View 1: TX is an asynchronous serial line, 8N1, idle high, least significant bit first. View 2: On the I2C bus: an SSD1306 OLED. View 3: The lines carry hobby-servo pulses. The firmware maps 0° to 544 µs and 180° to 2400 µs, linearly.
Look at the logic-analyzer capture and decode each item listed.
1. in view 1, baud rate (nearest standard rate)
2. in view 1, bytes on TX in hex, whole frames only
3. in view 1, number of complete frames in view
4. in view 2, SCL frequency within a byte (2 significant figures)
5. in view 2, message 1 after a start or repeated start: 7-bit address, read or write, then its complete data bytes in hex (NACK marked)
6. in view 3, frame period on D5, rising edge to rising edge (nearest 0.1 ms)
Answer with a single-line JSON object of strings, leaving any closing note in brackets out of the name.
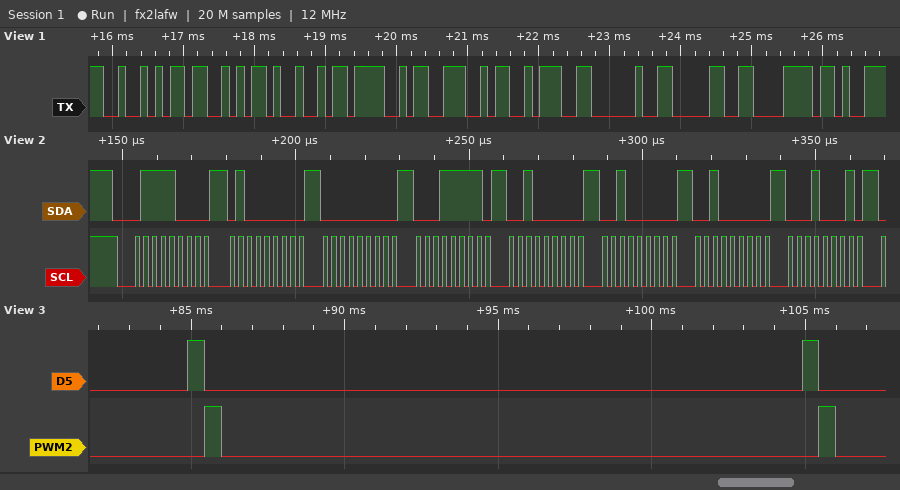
{"in view 1, baud rate": "9600 baud", "in view 1, bytes on TX in hex, whole frames only": "0x52 0x53 0x49 0x4F 0x4E 0x3A 0x20 0x30 0x78", "in view 1, number of complete frames in view": "9", "in view 2, SCL frequency within a byte": "400 kHz", "in view 2, message 1 after a start or repeated start: 7-bit address, read or write, then its complete data bytes in hex": "0x3C write: 40 00 1F 20 20 20 11", "in view 3, frame period on D5, rising edge to rising edge": "20.0 ms"}
